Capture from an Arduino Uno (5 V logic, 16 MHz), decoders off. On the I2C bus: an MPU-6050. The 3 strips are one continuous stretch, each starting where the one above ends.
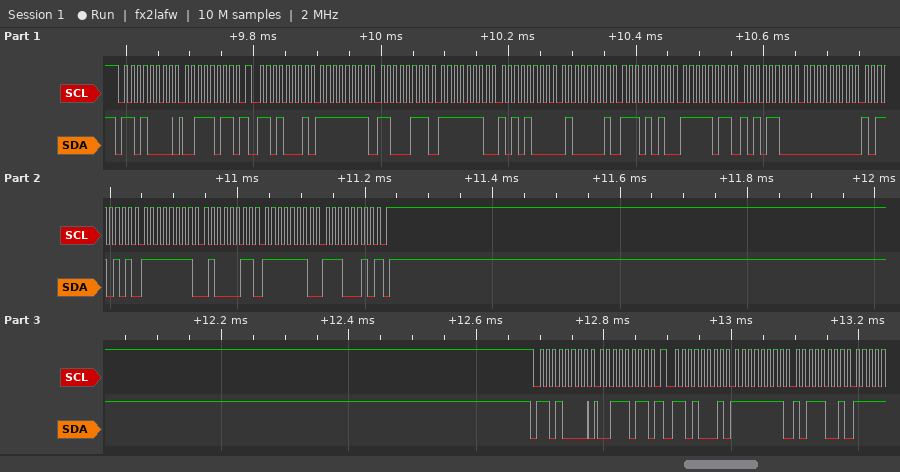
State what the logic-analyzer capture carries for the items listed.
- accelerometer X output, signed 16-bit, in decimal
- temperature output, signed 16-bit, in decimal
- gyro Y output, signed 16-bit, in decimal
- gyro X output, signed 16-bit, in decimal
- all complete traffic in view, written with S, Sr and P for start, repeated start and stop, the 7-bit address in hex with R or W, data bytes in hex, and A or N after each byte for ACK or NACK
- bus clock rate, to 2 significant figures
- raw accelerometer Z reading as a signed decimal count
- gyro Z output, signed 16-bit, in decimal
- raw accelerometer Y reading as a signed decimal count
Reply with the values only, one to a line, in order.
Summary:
-57
-1108
-189
181
S 68W A 3B A Sr 68R A FF A C7 A FE A A8 A 41 A EA A FB A AC A 00 A B5 A FF A 43 A FE A E2 N P S 68W A 3B A Sr 68R A FF A B9 A
100 kHz
16874
-286
-344
